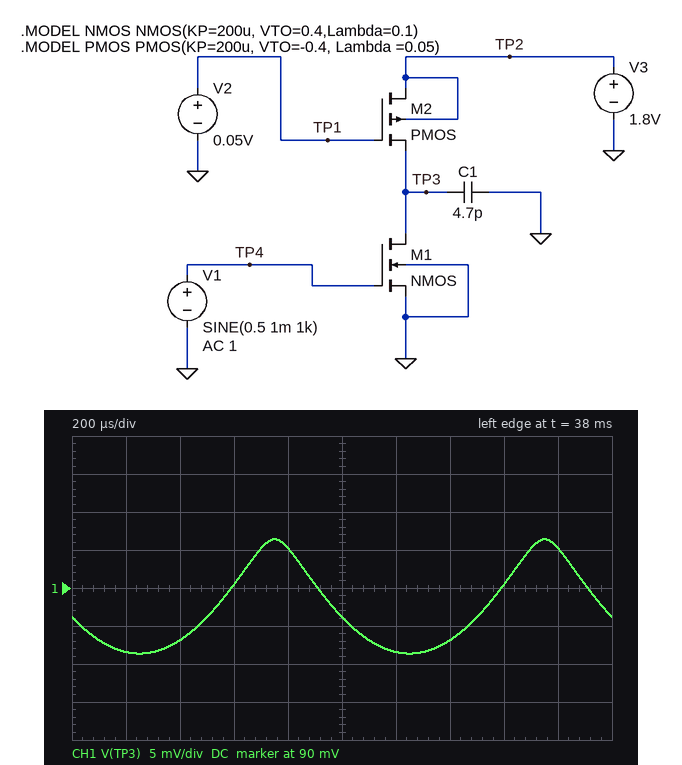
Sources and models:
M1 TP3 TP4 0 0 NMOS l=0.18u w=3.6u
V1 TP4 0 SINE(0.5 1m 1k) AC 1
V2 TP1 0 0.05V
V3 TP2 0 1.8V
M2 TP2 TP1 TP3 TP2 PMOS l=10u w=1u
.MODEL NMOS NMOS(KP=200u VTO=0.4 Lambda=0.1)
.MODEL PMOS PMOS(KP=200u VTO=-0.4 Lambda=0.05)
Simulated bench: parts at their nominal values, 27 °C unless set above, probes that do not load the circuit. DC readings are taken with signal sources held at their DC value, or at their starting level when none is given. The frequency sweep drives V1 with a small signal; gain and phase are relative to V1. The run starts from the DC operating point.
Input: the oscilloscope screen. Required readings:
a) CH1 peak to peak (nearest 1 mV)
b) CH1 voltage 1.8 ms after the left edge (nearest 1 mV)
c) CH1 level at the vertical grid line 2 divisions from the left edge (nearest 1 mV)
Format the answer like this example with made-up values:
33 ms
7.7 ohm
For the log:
15 mV
95 mV
83 mV
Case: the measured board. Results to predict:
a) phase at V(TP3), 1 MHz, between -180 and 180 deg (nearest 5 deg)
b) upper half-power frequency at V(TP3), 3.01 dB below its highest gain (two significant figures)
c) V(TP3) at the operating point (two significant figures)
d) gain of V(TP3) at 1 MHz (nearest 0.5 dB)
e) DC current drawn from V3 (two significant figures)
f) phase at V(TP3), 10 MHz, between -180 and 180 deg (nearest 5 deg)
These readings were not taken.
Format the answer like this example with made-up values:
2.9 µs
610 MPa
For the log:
155 deg
2.0 MHz
86 mV
14.5 dB
20 µA
100 deg
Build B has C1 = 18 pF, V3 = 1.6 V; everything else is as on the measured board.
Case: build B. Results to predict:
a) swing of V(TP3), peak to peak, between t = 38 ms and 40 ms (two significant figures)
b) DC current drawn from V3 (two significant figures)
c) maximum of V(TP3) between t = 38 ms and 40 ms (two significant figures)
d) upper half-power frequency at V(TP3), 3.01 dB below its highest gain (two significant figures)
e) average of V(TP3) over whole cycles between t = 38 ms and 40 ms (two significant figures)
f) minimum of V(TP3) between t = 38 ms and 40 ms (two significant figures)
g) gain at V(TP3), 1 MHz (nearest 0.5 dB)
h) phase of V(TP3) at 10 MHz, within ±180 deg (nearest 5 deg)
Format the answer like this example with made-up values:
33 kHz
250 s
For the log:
1.7 mV
14 µA
47 mV
1.9 MHz
46 mV
45 mV
-2.5 dB
100 deg
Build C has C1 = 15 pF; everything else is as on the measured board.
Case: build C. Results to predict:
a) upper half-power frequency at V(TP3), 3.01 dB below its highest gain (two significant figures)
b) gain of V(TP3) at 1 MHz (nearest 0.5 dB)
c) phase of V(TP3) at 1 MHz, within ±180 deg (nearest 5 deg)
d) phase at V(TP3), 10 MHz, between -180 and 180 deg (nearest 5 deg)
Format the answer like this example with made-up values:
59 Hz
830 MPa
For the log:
620 kHz
10.0 dB
120 deg
95 deg
